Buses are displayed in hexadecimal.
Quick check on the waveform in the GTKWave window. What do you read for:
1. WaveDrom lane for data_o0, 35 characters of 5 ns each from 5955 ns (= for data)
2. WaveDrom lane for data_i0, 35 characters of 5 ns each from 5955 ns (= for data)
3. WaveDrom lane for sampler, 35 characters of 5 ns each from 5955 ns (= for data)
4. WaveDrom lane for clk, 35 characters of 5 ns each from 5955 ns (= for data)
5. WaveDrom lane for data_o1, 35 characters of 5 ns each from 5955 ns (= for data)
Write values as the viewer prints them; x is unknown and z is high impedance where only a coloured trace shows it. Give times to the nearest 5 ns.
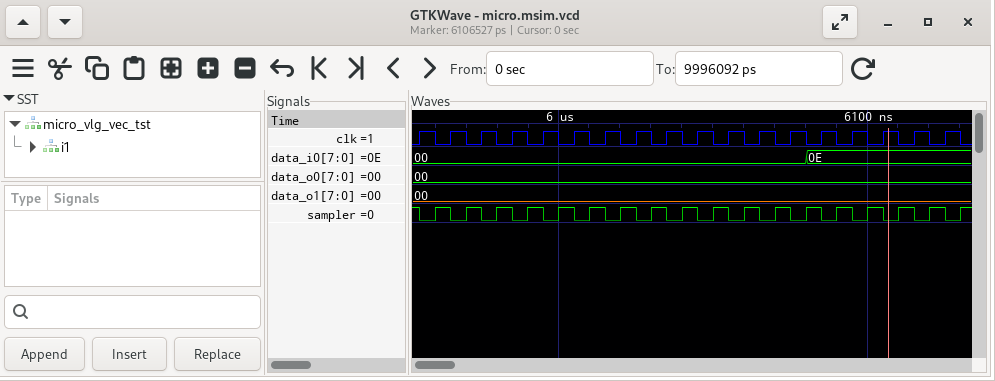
{name: 'data_o0', wave: '=..................................', data: '00'}
{name: 'data_i0', wave: '=........................=.........', data: '00 0E'}
{name: 'sampler', wave: '01010101010101010101010101010101010'}
{name: 'clk', wave: '10101010101010101010101010101010101'}
{name: 'data_o1', wave: '=..................................', data: '00'}
